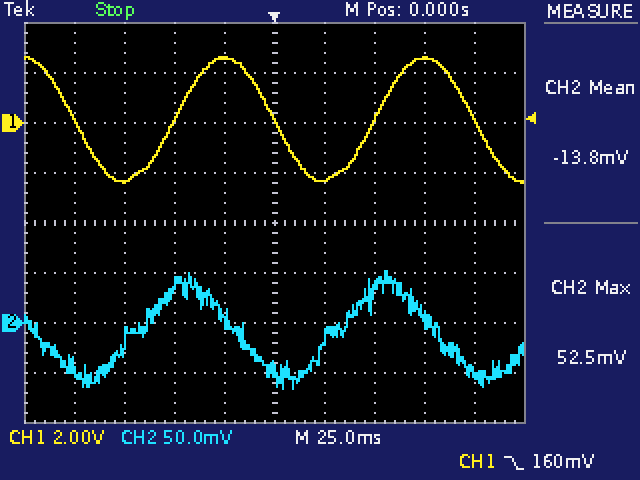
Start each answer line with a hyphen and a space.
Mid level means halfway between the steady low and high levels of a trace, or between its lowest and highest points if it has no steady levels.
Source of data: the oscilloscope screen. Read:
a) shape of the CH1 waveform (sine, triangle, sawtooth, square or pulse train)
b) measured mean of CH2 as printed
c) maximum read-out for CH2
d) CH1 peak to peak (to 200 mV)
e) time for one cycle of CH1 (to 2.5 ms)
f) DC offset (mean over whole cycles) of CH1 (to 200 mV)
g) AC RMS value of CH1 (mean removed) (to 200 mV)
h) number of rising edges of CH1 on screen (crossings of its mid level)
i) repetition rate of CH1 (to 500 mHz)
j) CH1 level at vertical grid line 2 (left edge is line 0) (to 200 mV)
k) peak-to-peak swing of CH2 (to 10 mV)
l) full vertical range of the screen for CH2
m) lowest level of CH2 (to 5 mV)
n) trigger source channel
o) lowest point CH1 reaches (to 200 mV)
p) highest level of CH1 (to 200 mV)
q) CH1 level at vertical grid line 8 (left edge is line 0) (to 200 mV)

- sine
- -13.8 mV
- 52.5 mV
- 5.0 V
- 100.0 ms
- 200 mV
- 1.8 V
- 2
- 10.0 Hz
- -2.4 V
- 120 mV
- 400 mV
- -65 mV
- CH1
- -2.4 V
- 2.6 V
- 2.6 V
